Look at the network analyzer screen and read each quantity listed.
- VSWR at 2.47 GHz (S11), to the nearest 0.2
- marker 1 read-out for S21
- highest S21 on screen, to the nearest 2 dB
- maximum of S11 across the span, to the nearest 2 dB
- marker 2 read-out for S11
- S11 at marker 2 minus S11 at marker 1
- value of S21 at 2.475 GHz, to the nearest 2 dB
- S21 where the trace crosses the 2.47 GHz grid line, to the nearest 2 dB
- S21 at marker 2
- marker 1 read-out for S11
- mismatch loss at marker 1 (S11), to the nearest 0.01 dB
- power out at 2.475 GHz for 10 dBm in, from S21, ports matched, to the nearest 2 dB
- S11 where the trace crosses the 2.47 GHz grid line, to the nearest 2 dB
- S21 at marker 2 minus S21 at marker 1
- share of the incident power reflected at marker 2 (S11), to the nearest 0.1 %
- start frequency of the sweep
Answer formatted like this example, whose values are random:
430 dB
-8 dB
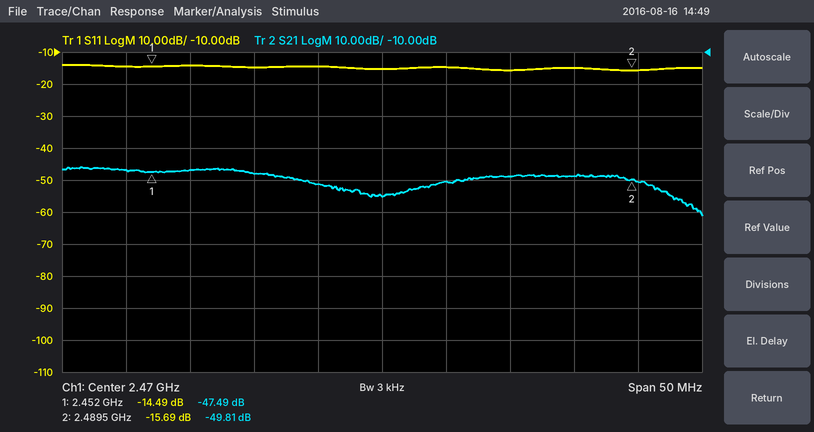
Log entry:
1.4
-47.49 dB
-46 dB
-14 dB
-15.69 dB
-1.20 dB
-50 dB
-56 dB
-49.81 dB
-14.49 dB
0.16 dB
-40 dBm
-16 dB
-2.32 dB
2.7 %
2.445 GHz
